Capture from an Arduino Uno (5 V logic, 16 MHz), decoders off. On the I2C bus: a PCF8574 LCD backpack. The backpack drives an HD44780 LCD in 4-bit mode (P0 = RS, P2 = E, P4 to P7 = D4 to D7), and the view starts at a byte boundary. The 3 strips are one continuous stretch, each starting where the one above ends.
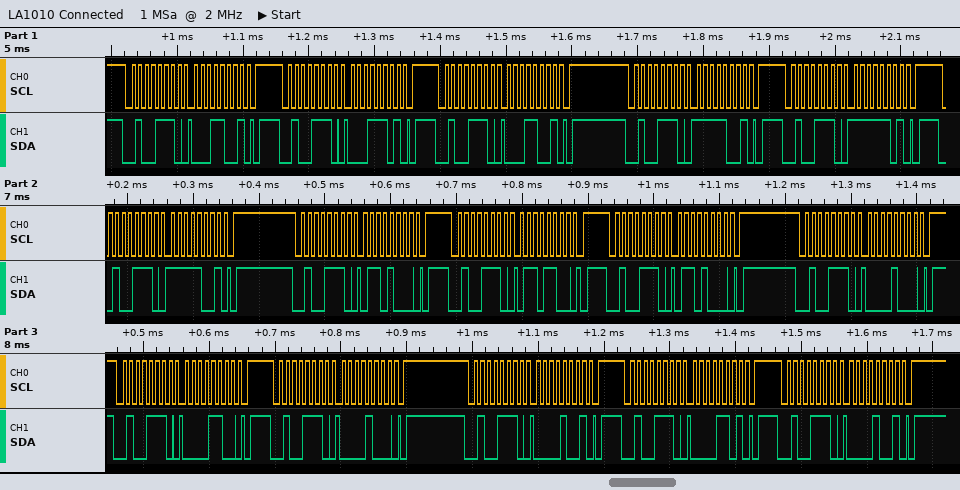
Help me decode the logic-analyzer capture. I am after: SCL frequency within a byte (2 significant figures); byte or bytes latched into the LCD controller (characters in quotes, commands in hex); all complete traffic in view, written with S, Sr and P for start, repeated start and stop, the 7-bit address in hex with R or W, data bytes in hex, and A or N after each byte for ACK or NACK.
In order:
100 kHz
data 0x1F 0x60
S 27W A 19 A P S 27W A 1D A P S 27W A 19 A P S 27W A F9 A P S 27W A FD A P S 27W A F9 A P S 27W A 68 A P S 27W A 6C A P S 27W A 68 A P S 27W A 08 A P S 27W A 0C A P S 27W A 08 A P S 27W A 09 A P S 27W A 0D A P S 27W A 09 A P
